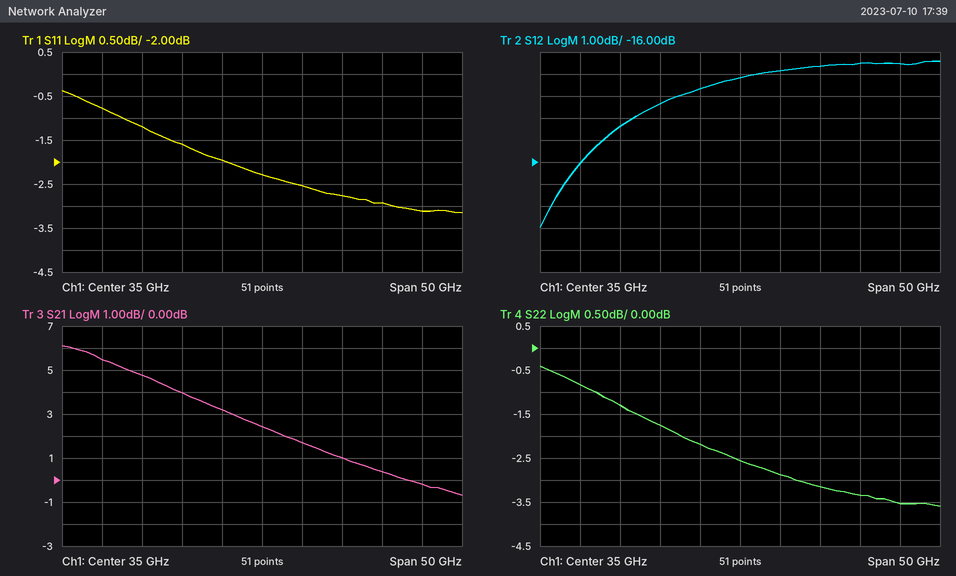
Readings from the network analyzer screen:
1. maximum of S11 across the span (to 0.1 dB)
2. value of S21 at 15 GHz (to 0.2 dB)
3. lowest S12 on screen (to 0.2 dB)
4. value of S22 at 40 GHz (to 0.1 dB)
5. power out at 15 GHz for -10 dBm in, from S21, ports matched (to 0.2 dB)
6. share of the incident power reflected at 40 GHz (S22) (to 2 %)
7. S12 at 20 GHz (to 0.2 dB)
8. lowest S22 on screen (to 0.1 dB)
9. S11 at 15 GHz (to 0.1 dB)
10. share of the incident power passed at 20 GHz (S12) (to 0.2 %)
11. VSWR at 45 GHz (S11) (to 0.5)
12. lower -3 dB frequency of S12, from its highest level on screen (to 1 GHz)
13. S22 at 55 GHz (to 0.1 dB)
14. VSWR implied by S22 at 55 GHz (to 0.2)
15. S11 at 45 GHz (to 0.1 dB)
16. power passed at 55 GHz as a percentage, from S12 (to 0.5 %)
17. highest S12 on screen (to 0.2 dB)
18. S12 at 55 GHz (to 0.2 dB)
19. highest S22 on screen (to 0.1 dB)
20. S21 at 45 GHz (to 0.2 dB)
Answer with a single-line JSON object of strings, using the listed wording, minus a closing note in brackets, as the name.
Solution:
{"maximum of S11 across the span": "-0.4 dB", "value of S21 at 15 GHz": "5.4 dB", "lowest S12 on screen": "-19.0 dB", "value of S22 at 40 GHz": "-2.9 dB", "power out at 15 GHz for -10 dBm in, from S21, ports matched": "-4.6 dBm", "share of the incident power reflected at 40 GHz (S22)": "52 %", "S12 at 20 GHz": "-14.4 dB", "lowest S22 on screen": "-3.6 dB", "S11 at 15 GHz": "-0.8 dB", "share of the incident power passed at 20 GHz (S12)": "3.6 %", "VSWR at 45 GHz (S11)": "6.5", "lower -3 dB frequency of S12, from its highest level on screen": "20 GHz", "S22 at 55 GHz": "-3.5 dB", "VSWR implied by S22 at 55 GHz": "5.0", "S11 at 45 GHz": "-2.8 dB", "power passed at 55 GHz as a percentage, from S12": "7.0 %", "highest S12 on screen": "-11.4 dB", "S12 at 55 GHz": "-11.6 dB", "highest S22 on screen": "-0.4 dB", "S21 at 45 GHz": "1.0 dB"}
